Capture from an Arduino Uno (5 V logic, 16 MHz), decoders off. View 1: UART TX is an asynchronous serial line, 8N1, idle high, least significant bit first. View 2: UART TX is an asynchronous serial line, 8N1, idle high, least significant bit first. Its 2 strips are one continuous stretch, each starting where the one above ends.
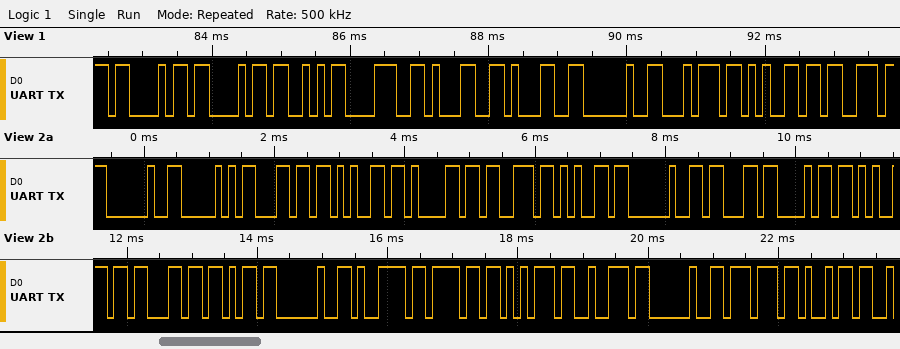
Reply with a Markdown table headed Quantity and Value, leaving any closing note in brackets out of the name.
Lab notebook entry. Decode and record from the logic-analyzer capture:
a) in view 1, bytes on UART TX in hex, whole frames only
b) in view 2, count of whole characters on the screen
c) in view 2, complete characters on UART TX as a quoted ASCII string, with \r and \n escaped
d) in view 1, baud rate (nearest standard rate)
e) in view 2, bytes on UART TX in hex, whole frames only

| Quantity | Value |
|---|---|
| in view 1, bytes on UART TX in hex, whole frames only | 0x43 0x43 0x53 0x38 0x31 0x31 0x20 0x74 0x65 0x73 |
| in view 2, count of whole characters on the screen | 21 |
| in view 2, complete characters on UART TX as a quoted ASCII string, with \r and \n escaped | " Please check your wi" |
| in view 1, baud rate | 9600 baud |
| in view 2, bytes on UART TX in hex, whole frames only | 0x20 0x50 0x6C 0x65 0x61 0x73 0x65 0x20 0x63 0x68 0x65 0x63 0x6B 0x20 0x79 0x6F 0x75 0x72 0x20 0x77 0x69 |
